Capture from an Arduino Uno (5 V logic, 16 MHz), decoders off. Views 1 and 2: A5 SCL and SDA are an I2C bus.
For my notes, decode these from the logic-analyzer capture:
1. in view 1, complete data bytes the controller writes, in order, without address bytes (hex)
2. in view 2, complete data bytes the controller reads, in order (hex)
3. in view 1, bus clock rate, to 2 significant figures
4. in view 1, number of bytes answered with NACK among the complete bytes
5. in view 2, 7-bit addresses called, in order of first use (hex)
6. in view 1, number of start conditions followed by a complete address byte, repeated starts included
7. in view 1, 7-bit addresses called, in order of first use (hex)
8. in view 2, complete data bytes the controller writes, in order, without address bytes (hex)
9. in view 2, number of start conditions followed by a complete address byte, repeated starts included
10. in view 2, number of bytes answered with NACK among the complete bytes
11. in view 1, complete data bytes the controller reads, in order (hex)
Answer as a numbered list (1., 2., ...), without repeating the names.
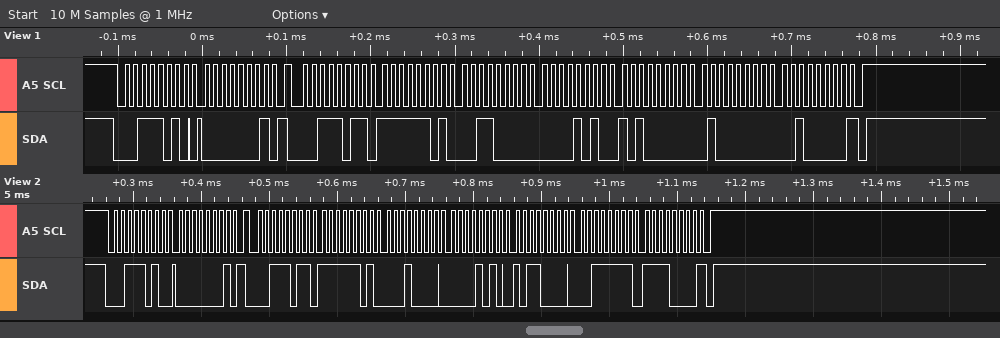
1. 01
2. FD 10 0A B0 3F F0
3. 100 kHz
4. 1
5. 0x1D
6. 2
7. 0x1D
8. 01
9. 2
10. 1
11. FD 30 0A A0 40 20
